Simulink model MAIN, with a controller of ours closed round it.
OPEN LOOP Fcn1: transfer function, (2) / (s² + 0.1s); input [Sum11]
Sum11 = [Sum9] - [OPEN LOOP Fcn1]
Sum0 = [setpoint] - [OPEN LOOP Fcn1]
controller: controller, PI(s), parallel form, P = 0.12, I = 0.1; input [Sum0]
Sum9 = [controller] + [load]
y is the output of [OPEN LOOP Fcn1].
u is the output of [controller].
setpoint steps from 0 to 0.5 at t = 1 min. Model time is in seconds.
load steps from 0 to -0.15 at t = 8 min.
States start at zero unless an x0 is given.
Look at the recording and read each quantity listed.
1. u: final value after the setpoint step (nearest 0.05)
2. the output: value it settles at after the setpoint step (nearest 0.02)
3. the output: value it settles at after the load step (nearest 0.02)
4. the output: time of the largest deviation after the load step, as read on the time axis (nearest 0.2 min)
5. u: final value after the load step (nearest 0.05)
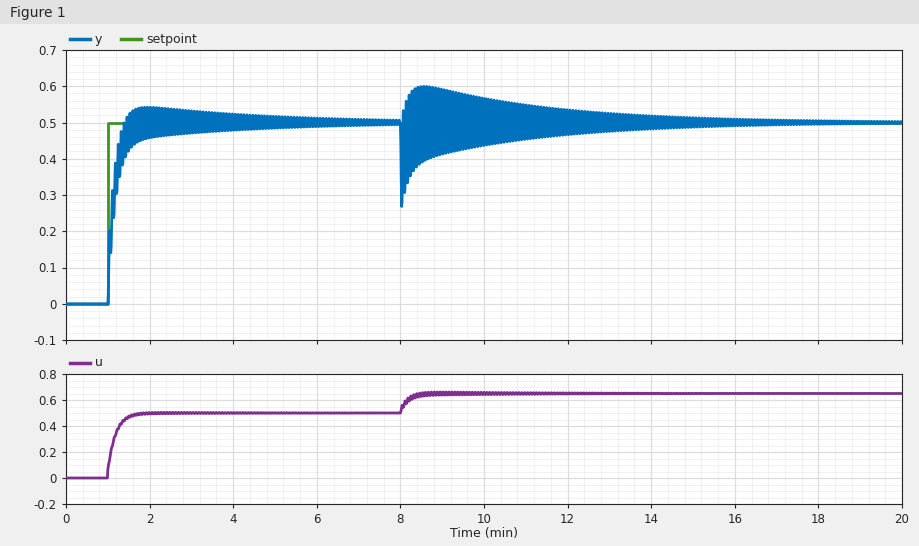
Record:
0.50
0.50
0.50
8.0 min
0.65
